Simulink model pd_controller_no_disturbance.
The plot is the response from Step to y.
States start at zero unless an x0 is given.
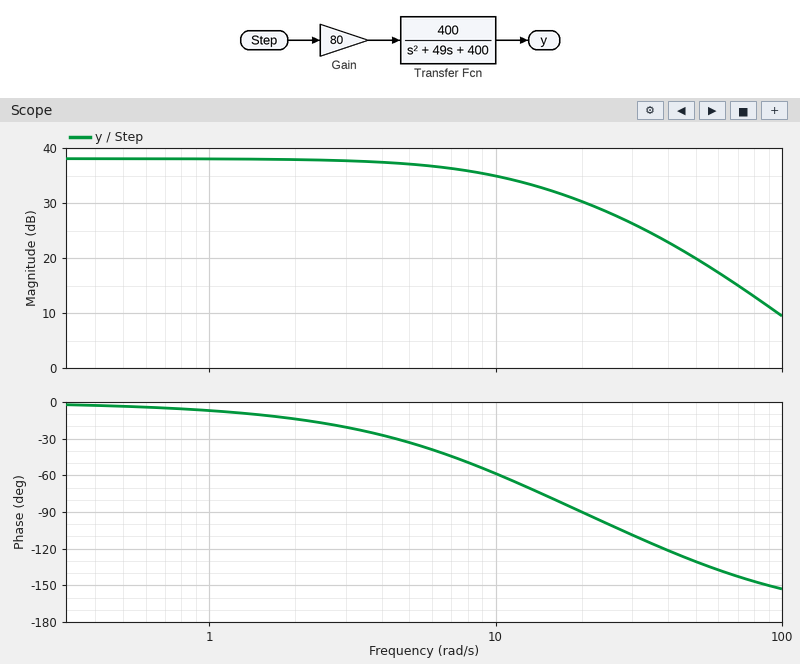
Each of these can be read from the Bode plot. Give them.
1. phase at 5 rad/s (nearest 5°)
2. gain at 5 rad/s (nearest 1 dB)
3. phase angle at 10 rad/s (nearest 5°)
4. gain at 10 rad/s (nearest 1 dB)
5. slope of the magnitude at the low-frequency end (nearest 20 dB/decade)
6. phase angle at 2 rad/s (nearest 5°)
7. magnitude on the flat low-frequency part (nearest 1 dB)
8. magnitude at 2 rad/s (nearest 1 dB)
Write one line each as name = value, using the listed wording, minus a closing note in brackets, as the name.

phase at 5 rad/s = -35°
gain at 5 rad/s = 37 dB
phase angle at 10 rad/s = -60°
gain at 10 rad/s = 35 dB
slope of the magnitude at the low-frequency end = 0 dB/decade
phase angle at 2 rad/s = -15°
magnitude on the flat low-frequency part = 38 dB
magnitude at 2 rad/s = 38 dB
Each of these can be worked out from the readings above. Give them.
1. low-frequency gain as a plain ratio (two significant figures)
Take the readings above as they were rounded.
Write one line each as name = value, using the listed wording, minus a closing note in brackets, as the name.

low-frequency gain as a plain ratio = 79
